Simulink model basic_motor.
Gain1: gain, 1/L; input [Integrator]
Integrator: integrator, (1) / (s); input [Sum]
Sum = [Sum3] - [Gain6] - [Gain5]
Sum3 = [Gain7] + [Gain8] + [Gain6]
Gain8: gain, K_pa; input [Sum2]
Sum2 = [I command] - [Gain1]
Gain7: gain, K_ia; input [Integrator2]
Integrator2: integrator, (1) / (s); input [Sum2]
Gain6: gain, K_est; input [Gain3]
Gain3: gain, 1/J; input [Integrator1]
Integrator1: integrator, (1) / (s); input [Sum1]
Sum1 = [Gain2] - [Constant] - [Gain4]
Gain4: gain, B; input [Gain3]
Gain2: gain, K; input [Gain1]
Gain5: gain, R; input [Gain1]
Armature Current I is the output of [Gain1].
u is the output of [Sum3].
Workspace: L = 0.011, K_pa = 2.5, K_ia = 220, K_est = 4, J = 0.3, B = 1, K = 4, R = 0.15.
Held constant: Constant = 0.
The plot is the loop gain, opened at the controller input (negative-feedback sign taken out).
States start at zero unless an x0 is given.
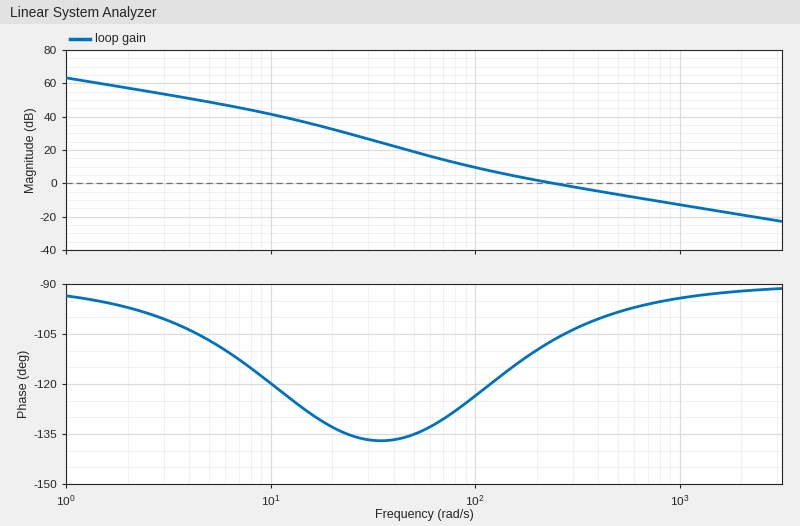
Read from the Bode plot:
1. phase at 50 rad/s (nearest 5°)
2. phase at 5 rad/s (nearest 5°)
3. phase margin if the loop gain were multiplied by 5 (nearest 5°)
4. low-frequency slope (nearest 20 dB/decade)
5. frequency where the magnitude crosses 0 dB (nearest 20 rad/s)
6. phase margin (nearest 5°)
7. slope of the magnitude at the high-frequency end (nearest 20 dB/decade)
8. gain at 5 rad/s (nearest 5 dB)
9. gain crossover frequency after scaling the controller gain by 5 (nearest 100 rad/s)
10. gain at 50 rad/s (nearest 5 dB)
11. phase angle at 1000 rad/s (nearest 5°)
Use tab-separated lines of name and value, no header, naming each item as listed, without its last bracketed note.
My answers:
phase at 50 rad/s	-135°
phase at 5 rad/s	-105°
phase margin if the loop gain were multiplied by 5	85°
low-frequency slope	-20 dB/decade
frequency where the magnitude crosses 0 dB	240 rad/s
phase margin	75°
slope of the magnitude at the high-frequency end	-20 dB/decade
gain at 5 rad/s	50 dB
gain crossover frequency after scaling the controller gain by 5	1100 rad/s
gain at 50 rad/s	20 dB
phase angle at 1000 rad/s	-95°
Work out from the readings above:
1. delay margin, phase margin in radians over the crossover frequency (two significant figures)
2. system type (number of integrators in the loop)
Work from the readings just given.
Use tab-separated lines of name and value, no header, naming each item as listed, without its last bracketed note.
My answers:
delay margin, phase margin in radians over the crossover frequency	0.0055 s
system type	1
